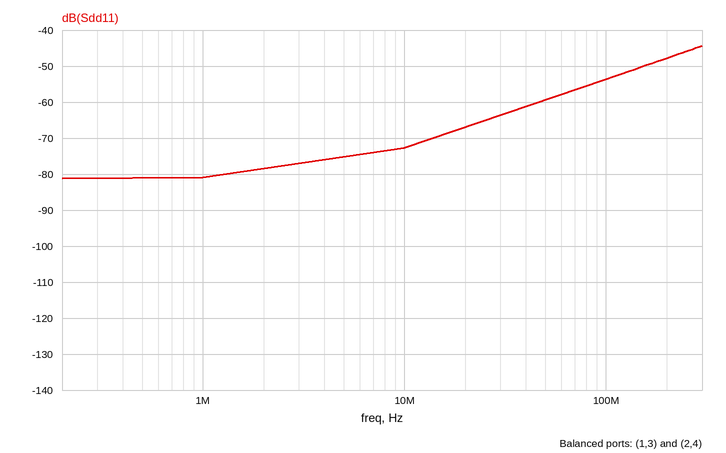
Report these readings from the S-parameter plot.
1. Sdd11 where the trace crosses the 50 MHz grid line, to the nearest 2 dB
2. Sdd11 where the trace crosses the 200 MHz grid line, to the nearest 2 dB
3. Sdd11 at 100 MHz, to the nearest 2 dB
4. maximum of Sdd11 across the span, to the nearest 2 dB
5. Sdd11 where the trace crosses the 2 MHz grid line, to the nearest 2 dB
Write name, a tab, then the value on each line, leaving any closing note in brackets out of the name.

Sdd11 where the trace crosses the 50 MHz grid line, to the nearest 2 dB	-60 dB
Sdd11 where the trace crosses the 200 MHz grid line, to the nearest 2 dB	-48 dB
Sdd11 at 100 MHz, to the nearest 2 dB	-54 dB
maximum of Sdd11 across the span, to the nearest 2 dB	-44 dB
Sdd11 where the trace crosses the 2 MHz grid line, to the nearest 2 dB	-78 dB
